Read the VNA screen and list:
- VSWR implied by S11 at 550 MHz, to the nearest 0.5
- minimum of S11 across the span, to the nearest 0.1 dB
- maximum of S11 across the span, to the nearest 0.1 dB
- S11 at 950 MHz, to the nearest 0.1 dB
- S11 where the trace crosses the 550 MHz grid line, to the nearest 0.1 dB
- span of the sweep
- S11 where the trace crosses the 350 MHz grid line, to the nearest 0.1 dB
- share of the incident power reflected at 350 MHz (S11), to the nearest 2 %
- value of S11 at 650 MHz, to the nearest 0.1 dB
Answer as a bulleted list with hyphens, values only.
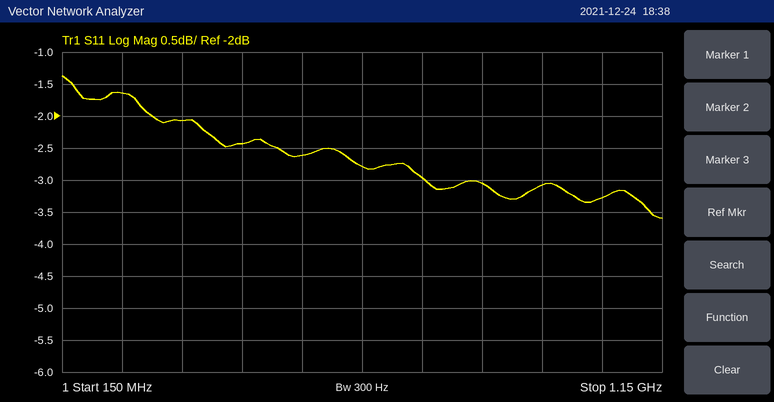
- 6.5
- -3.6 dB
- -1.4 dB
- -3.1 dB
- -2.6 dB
- 1 GHz
- -2.1 dB
- 62 %
- -2.8 dB
